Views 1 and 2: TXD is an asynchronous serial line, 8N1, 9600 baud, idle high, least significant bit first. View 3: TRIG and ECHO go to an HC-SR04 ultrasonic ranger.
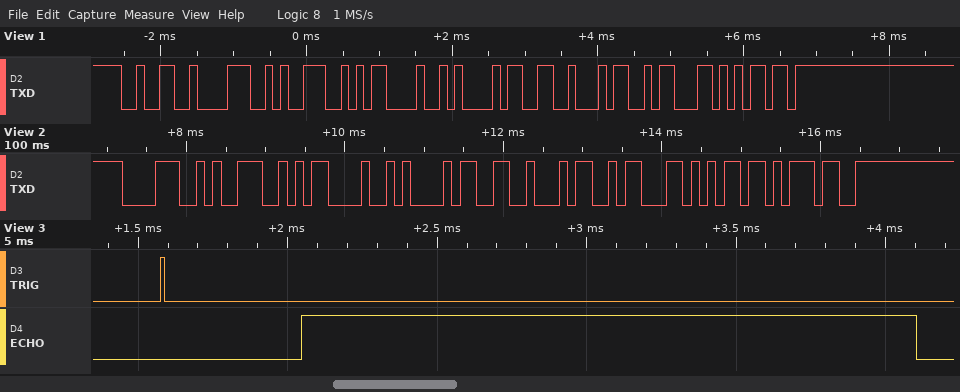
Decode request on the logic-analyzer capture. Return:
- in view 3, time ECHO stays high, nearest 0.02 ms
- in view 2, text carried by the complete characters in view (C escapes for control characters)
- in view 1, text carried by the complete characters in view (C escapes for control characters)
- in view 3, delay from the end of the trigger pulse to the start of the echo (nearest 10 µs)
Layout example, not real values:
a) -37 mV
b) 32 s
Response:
a) 2.06 ms
b) "89\r\n34cm7"
c) "289\r\n34cm"
d) 460 µs
